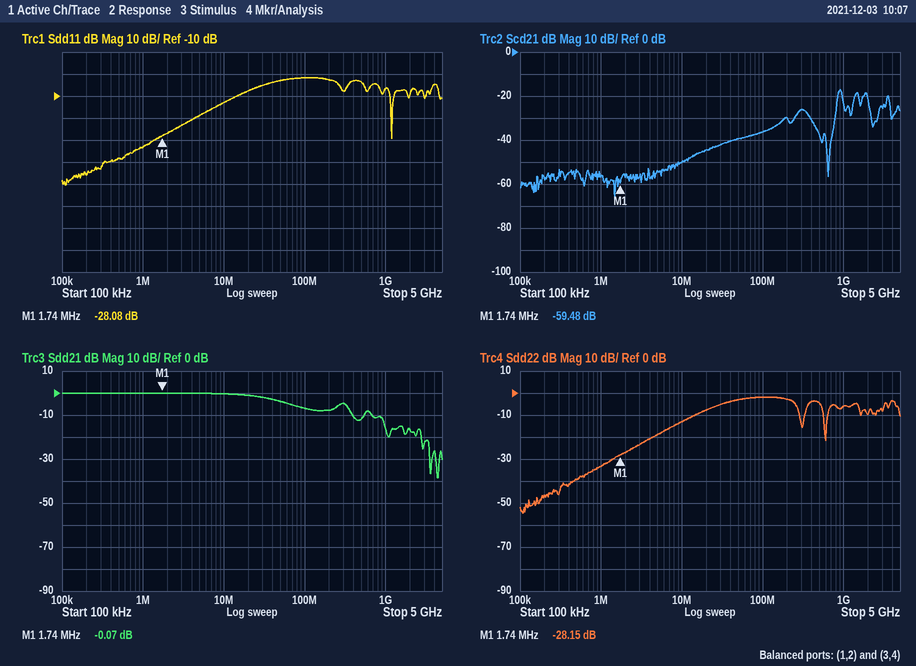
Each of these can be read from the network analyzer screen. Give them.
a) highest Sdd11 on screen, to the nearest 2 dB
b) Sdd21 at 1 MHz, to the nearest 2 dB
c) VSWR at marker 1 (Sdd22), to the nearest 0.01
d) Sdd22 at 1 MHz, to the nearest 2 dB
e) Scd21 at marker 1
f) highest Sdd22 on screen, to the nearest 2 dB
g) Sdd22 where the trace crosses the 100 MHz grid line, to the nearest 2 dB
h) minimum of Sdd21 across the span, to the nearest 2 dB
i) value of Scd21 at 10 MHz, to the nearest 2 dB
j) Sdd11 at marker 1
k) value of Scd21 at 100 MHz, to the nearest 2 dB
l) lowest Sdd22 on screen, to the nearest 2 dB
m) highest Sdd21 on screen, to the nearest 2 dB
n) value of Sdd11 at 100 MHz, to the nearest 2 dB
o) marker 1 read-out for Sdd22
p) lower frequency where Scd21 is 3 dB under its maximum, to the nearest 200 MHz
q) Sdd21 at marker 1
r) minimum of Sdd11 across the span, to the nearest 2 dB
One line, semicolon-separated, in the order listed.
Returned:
-2 dB; 0 dB; 1.08; -34 dB; -59.48 dB; -2 dB; -2 dB; -38 dB; -50 dB; -28.08 dB; -36 dB; -54 dB; 0 dB; -2 dB; -28.15 dB; 800 MHz; -0.07 dB; -50 dB
